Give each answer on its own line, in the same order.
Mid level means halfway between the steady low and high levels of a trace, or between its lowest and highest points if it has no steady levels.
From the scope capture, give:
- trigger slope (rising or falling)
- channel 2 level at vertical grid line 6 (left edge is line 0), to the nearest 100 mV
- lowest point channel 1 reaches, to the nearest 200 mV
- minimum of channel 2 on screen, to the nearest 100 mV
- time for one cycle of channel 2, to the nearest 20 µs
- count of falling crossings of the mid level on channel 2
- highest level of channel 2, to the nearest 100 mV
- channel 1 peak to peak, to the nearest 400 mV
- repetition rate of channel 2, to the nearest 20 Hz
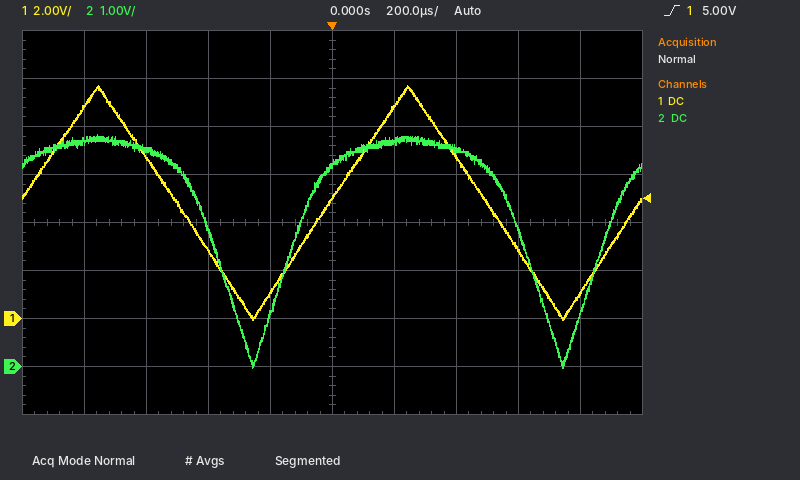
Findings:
rising
4.7 V
0.0 V
0.0 V
1.00 ms
2
4.8 V
9.6 V
1.00 kHz
